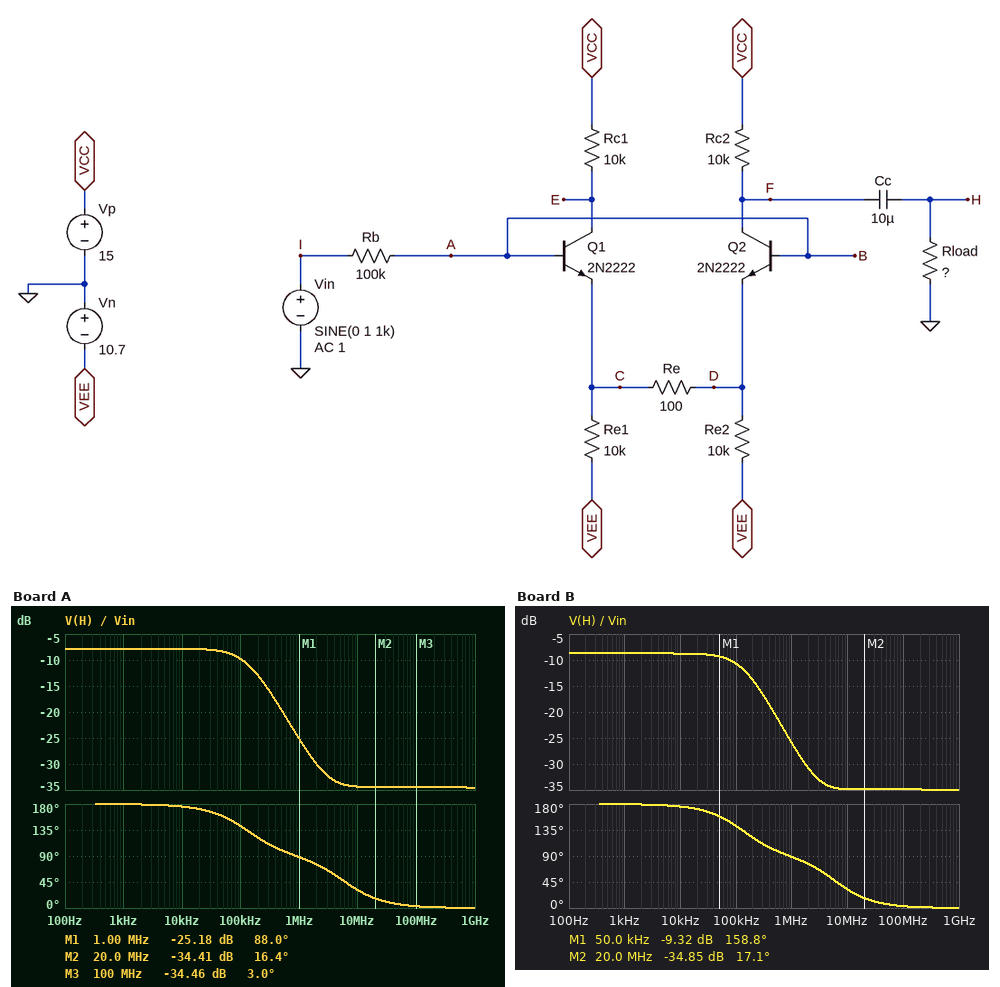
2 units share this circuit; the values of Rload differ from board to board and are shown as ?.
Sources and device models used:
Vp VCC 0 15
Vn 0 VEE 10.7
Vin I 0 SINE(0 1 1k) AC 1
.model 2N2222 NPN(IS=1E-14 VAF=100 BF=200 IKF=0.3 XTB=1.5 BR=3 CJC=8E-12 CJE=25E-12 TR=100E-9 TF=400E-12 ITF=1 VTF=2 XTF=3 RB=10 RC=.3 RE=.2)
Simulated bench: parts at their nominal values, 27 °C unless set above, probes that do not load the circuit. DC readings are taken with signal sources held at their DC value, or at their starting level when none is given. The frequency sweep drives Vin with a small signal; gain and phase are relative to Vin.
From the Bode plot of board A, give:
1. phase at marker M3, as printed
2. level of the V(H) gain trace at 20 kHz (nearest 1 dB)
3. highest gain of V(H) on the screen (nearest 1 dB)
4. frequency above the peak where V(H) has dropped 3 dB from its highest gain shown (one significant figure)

3.0 deg
-8 dB
-8 dB
100 kHz
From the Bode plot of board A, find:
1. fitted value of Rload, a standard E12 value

8.2 kΩ
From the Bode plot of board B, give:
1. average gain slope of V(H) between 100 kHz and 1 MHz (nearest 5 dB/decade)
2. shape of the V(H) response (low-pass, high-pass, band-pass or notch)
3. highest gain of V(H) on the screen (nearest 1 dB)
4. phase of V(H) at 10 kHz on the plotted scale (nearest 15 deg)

-15 dB/decade
low-pass
-9 dB
180 deg
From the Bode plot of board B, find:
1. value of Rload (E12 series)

6.8 kΩ
